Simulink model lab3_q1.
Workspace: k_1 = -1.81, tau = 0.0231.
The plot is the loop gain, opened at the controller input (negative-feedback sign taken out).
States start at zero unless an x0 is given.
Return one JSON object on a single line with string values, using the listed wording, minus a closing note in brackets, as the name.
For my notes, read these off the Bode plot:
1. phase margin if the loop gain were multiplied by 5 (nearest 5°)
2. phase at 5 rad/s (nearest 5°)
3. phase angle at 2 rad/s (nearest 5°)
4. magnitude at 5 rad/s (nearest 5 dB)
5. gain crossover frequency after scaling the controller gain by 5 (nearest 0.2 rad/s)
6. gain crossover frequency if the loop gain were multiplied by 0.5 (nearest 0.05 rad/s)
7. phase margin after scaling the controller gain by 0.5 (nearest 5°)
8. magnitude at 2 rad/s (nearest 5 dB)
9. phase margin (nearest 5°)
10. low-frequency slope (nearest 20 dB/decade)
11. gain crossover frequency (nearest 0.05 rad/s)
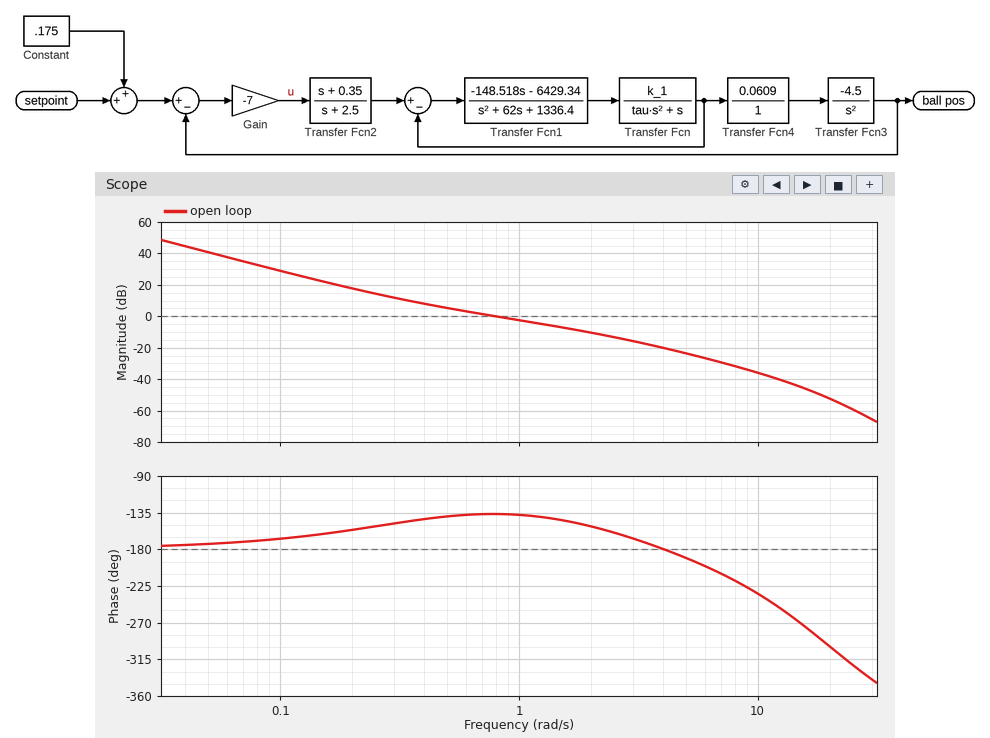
{"phase margin if the loop gain were multiplied by 5": "20°", "phase at 5 rad/s": "-190°", "phase angle at 2 rad/s": "-150°", "magnitude at 5 rad/s": "-25 dB", "gain crossover frequency after scaling the controller gain by 5": "2.6 rad/s", "gain crossover frequency if the loop gain were multiplied by 0.5": "0.45 rad/s", "phase margin after scaling the controller gain by 0.5": "40°", "magnitude at 2 rad/s": "-10 dB", "phase margin": "45°", "low-frequency slope": "-40 dB/decade", "gain crossover frequency": "0.80 rad/s"}
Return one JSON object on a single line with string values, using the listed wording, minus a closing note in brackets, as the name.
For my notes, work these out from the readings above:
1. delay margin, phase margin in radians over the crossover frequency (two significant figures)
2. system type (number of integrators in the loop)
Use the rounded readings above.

{"delay margin, phase margin in radians over the crossover frequency": "0.98 s", "system type": "2"}
